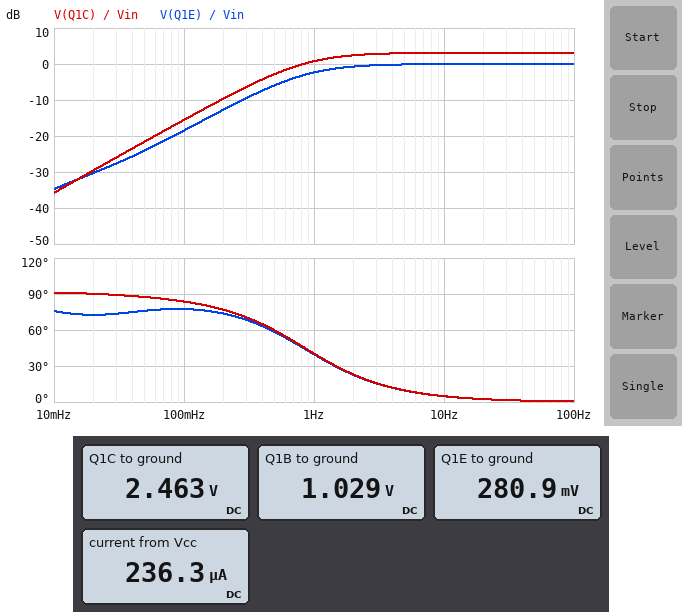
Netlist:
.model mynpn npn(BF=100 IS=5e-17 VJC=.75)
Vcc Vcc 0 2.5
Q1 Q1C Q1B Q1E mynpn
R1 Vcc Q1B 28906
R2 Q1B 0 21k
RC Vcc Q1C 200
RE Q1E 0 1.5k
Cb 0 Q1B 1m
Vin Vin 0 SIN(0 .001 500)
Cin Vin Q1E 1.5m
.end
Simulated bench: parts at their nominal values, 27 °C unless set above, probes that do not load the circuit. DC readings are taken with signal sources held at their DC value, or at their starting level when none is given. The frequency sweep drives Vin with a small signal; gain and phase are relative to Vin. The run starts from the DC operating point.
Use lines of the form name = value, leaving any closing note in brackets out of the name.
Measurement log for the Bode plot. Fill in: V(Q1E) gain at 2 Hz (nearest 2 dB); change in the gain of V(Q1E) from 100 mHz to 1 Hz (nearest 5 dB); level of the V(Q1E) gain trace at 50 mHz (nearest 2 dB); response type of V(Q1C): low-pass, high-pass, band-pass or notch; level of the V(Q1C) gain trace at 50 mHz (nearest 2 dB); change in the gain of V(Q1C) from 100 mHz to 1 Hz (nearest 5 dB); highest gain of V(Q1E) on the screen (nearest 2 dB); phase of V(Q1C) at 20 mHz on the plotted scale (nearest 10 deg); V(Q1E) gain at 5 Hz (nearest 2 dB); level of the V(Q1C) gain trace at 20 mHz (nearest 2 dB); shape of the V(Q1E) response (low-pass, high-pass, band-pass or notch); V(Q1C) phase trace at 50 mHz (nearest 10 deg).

V(Q1E) gain at 2 Hz = 0 dB
change in the gain of V(Q1E) from 100 mHz to 1 Hz = 15 dB
level of the V(Q1E) gain trace at 50 mHz = -24 dB
response type of V(Q1C): low-pass, high-pass, band-pass or notch = high-pass
level of the V(Q1C) gain trace at 50 mHz = -22 dB
change in the gain of V(Q1C) from 100 mHz to 1 Hz = 15 dB
highest gain of V(Q1E) on the screen = 0 dB
phase of V(Q1C) at 20 mHz on the plotted scale = 90 deg
V(Q1E) gain at 5 Hz = 0 dB
level of the V(Q1C) gain trace at 20 mHz = -30 dB
shape of the V(Q1E) response = high-pass
V(Q1C) phase trace at 50 mHz = 90 deg
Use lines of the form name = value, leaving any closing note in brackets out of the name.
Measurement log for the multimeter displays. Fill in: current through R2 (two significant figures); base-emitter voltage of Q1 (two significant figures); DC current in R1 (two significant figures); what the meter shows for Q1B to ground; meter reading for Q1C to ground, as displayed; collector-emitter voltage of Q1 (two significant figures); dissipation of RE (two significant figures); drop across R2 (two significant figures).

current through R2 = 49 µA
base-emitter voltage of Q1 = 750 mV
DC current in R1 = 51 µA
what the meter shows for Q1B to ground = 1.029 V
meter reading for Q1C to ground, as displayed = 2.463 V
collector-emitter voltage of Q1 = 2.2 V
dissipation of RE = 53 µW
drop across R2 = 1.0 V
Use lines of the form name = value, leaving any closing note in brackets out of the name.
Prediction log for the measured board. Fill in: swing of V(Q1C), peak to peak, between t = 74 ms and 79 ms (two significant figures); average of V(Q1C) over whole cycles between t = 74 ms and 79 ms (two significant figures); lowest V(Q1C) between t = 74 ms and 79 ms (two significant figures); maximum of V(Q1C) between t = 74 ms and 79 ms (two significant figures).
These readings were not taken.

swing of V(Q1C), peak to peak, between t = 74 ms and 79 ms = 2.9 mV
average of V(Q1C) over whole cycles between t = 74 ms and 79 ms = 2.5 V
lowest V(Q1C) between t = 74 ms and 79 ms = 2.5 V
maximum of V(Q1C) between t = 74 ms and 79 ms = 2.5 V
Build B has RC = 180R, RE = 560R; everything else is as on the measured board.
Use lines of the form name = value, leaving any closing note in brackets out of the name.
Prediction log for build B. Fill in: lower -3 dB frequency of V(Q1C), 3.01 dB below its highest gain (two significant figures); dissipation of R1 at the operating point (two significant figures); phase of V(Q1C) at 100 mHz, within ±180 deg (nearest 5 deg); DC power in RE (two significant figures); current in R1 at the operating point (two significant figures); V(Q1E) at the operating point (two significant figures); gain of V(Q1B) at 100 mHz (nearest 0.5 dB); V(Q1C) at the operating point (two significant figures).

lower -3 dB frequency of V(Q1C), 3.01 dB below its highest gain = 1.9 Hz
dissipation of R1 at the operating point = 78 µW
phase of V(Q1C) at 100 mHz, within ±180 deg = 90 deg
DC power in RE = 97 µW
current in R1 at the operating point = 52 µA
V(Q1E) at the operating point = 230 mV
gain of V(Q1B) at 100 mHz = -37.5 dB
V(Q1C) at the operating point = 2.4 V
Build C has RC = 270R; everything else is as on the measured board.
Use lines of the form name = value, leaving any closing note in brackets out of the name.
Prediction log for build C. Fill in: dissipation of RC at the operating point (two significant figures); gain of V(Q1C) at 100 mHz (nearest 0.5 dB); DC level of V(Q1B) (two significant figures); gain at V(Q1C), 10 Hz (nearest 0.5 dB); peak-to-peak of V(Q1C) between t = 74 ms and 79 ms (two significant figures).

dissipation of RC at the operating point = 9.3 µW
gain of V(Q1C) at 100 mHz = -13.0 dB
DC level of V(Q1B) = 1.0 V
gain at V(Q1C), 10 Hz = 5.5 dB
peak-to-peak of V(Q1C) between t = 74 ms and 79 ms = 3.9 mV
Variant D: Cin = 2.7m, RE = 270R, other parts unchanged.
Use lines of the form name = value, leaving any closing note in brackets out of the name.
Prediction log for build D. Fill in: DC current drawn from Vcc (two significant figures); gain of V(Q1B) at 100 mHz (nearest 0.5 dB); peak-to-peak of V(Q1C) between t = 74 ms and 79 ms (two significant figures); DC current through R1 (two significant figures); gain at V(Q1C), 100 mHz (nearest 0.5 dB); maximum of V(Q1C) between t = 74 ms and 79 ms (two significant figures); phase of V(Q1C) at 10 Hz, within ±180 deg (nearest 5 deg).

DC current drawn from Vcc = 740 µA
gain of V(Q1B) at 100 mHz = -33.0 dB
peak-to-peak of V(Q1C) between t = 74 ms and 79 ms = 11 mV
DC current through R1 = 53 µA
gain at V(Q1C), 100 mHz = -11.0 dB
maximum of V(Q1C) between t = 74 ms and 79 ms = 2.4 V
phase of V(Q1C) at 10 Hz, within ±180 deg = 10 deg
